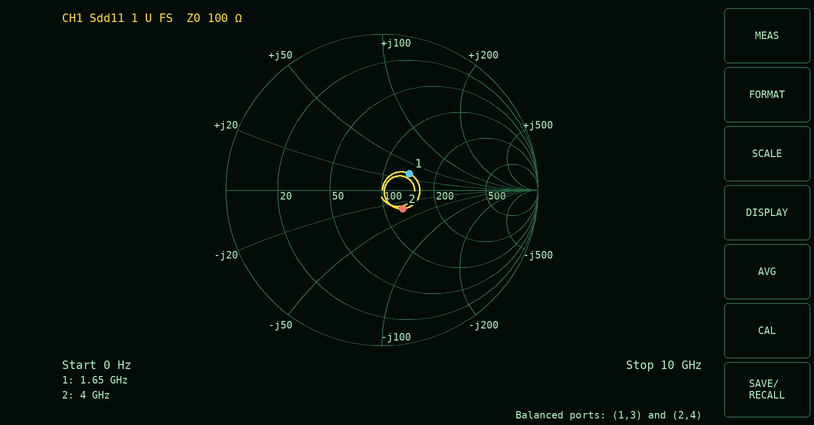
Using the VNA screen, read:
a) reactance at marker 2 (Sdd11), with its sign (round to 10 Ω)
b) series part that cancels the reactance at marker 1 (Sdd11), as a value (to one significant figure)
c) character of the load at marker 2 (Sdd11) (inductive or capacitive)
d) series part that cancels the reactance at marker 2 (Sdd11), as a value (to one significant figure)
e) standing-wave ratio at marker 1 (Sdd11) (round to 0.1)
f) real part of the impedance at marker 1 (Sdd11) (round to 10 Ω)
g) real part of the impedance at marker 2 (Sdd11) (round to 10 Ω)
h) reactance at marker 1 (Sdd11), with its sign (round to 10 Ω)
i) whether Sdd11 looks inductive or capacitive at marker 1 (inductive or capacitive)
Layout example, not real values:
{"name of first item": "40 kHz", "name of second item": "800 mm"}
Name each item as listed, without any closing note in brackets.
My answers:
{"reactance at marker 2 (Sdd11), with its sign": "-30 Ω", "series part that cancels the reactance at marker 1 (Sdd11), as a value": "3 pF", "character of the load at marker 2 (Sdd11)": "capacitive", "series part that cancels the reactance at marker 2 (Sdd11), as a value": "1 nH", "standing-wave ratio at marker 1 (Sdd11)": "1.5", "real part of the impedance at marker 1 (Sdd11)": "140 Ω", "real part of the impedance at marker 2 (Sdd11)": "130 Ω", "reactance at marker 1 (Sdd11), with its sign": "+30 Ω", "whether Sdd11 looks inductive or capacitive at marker 1": "inductive"}
